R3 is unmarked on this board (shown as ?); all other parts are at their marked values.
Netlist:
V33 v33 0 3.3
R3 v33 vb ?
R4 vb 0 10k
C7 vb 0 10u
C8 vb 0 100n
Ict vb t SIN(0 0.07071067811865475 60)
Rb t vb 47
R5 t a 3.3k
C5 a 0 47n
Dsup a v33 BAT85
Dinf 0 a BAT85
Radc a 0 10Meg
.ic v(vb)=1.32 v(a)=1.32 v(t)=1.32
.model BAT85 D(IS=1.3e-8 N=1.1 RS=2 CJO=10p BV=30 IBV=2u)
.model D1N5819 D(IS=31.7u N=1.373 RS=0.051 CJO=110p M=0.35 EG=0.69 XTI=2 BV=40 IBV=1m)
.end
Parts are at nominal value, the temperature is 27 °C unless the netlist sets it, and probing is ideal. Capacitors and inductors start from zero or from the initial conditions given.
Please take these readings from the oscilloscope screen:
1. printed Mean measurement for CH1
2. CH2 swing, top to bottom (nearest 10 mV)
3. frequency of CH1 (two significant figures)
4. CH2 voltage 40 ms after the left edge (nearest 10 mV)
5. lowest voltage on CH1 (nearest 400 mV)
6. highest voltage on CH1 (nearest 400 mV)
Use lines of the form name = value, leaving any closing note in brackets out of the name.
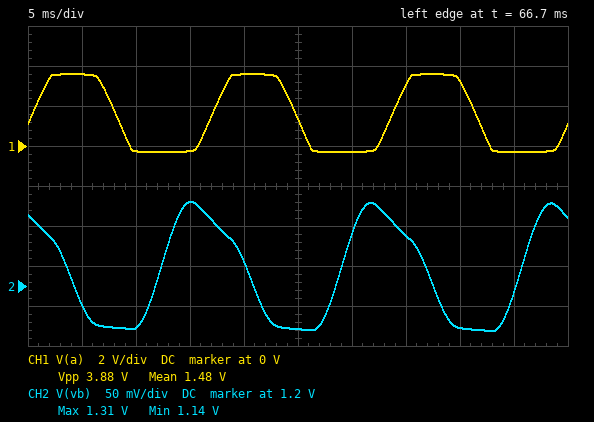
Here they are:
printed Mean measurement for CH1 = 1.48 V
CH2 swing, top to bottom = 160 mV
frequency of CH1 = 60 Hz
CH2 voltage 40 ms after the left edge = 1.15 V
lowest voltage on CH1 = -400 mV
highest voltage on CH1 = 3.6 V
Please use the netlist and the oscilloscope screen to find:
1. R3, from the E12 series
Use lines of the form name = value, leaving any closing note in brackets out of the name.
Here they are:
R3, from the E12 series = 47 kΩ
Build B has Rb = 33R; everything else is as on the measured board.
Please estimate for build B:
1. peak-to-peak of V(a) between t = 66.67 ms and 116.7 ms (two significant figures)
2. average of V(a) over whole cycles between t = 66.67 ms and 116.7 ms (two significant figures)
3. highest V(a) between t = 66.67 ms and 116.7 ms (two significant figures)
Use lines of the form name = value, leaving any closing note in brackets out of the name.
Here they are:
peak-to-peak of V(a) between t = 66.67 ms and 116.7 ms = 3.7 V
average of V(a) over whole cycles between t = 66.67 ms and 116.7 ms = 1.3 V
highest V(a) between t = 66.67 ms and 116.7 ms = 3.4 V
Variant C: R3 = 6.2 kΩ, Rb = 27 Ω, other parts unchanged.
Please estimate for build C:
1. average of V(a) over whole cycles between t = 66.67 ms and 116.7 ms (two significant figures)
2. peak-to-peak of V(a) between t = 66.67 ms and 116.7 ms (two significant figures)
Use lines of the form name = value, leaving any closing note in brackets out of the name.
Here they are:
average of V(a) over whole cycles between t = 66.67 ms and 116.7 ms = 1.9 V
peak-to-peak of V(a) between t = 66.67 ms and 116.7 ms = 3.5 V
